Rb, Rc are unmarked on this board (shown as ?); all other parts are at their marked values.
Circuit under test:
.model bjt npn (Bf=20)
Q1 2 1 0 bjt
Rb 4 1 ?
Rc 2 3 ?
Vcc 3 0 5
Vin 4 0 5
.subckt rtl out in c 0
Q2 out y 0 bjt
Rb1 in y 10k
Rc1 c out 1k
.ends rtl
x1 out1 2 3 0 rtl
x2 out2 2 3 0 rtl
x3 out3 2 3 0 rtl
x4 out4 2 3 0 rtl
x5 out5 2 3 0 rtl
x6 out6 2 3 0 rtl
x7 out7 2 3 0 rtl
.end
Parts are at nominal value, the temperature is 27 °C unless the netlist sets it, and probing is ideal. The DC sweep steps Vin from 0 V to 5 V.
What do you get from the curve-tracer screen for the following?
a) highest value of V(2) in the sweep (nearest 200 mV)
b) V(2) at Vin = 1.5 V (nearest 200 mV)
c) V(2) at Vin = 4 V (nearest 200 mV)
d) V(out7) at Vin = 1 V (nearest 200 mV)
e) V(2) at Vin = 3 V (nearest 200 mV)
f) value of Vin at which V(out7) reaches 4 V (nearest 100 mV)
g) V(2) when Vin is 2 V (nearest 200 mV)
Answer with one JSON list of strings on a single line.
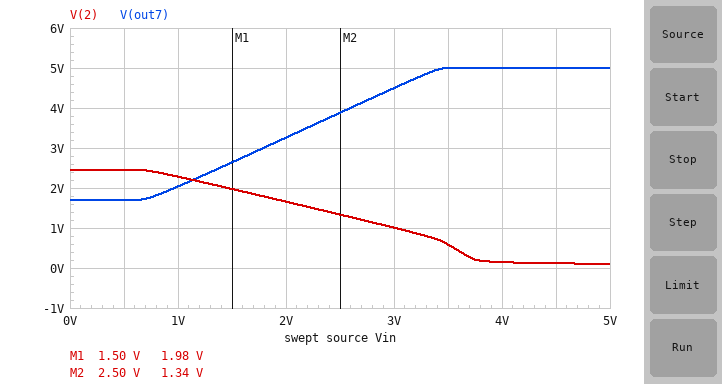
["2.4 V", "2.0 V", "200 mV", "2.0 V", "1.0 V", "2.6 V", "1.6 V"]
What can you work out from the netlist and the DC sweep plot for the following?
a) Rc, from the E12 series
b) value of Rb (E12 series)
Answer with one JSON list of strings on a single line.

["2.2 kΩ", "27 kΩ"]
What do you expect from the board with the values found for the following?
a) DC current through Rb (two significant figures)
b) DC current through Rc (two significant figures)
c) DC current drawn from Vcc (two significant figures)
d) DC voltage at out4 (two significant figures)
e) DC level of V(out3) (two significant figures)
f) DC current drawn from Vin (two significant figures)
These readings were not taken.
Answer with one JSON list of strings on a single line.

["160 µA", "2.2 mA", "2.2 mA", "5.0 V", "5.0 V", "160 µA"]
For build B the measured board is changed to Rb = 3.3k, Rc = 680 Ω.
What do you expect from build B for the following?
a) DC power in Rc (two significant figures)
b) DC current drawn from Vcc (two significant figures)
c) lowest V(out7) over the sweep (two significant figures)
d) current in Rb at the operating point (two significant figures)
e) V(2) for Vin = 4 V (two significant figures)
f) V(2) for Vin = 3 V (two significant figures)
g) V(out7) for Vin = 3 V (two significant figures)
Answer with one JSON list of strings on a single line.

["36 mW", "7.3 mA", "130 mV", "1.3 mA", "71 mV", "87 mV", "5.0 V"]
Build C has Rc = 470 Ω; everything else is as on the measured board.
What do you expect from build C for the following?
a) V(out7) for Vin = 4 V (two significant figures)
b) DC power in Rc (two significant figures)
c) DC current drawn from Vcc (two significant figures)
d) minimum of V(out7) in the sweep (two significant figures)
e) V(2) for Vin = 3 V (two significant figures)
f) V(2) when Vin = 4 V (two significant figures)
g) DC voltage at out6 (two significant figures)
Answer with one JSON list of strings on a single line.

["380 mV", "9.7 mW", "33 mA", "110 mV", "3.4 V", "3.1 V", "890 mV"]
